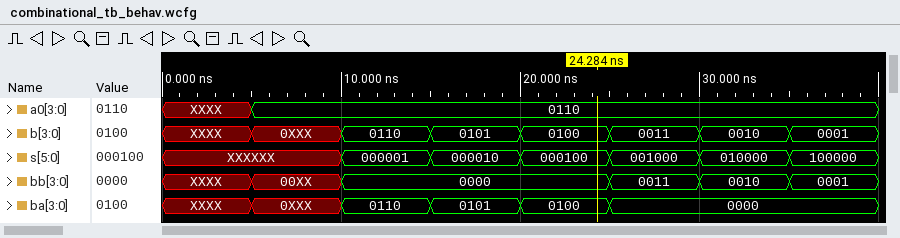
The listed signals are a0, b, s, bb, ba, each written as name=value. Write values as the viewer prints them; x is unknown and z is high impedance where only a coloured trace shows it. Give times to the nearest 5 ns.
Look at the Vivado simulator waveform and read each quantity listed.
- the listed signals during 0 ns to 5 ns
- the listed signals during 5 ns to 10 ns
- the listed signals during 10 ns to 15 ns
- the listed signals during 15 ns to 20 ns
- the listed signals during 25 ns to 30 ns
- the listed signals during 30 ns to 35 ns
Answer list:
a0=XXXX, b=XXXX, s=XXXXXX, bb=XXXX, ba=XXXX
a0=0110, b=0XXX, s=XXXXXX, bb=00XX, ba=0XXX
a0=0110, b=0110, s=000001, bb=0000, ba=0110
a0=0110, b=0101, s=000010, bb=0000, ba=0101
a0=0110, b=0011, s=001000, bb=0011, ba=0000
a0=0110, b=0010, s=010000, bb=0010, ba=0000
